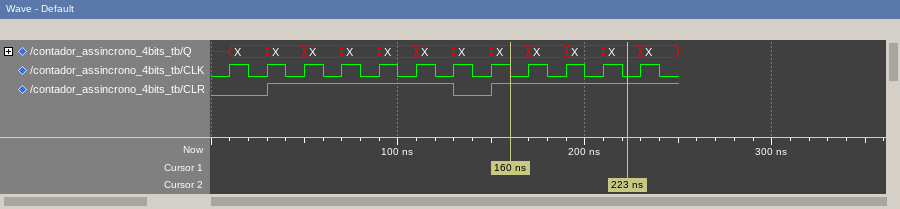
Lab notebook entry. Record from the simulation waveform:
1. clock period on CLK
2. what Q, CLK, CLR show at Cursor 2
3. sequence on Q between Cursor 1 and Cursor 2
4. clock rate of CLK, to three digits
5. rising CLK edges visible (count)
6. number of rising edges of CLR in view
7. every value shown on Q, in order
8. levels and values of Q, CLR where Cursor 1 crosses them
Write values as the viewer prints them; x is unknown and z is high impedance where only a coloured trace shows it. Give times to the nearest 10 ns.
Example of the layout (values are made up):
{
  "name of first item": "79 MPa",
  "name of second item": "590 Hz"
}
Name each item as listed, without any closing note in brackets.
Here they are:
{
  "clock period on CLK": "20 ns",
  "what Q, CLK, CLR show at Cursor 2": "Q=X, CLK=0, CLR=1",
  "sequence on Q between Cursor 1 and Cursor 2": "X, X, X, X",
  "clock rate of CLK, to three digits": "50.0 MHz",
  "rising CLK edges visible": "12",
  "number of rising edges of CLR in view": "2",
  "every value shown on Q, in order": "x, X, X, X, X, X, X, X, X, X, X, X, X",
  "levels and values of Q, CLR where Cursor 1 crosses them": "Q=X, CLR=1"
}
